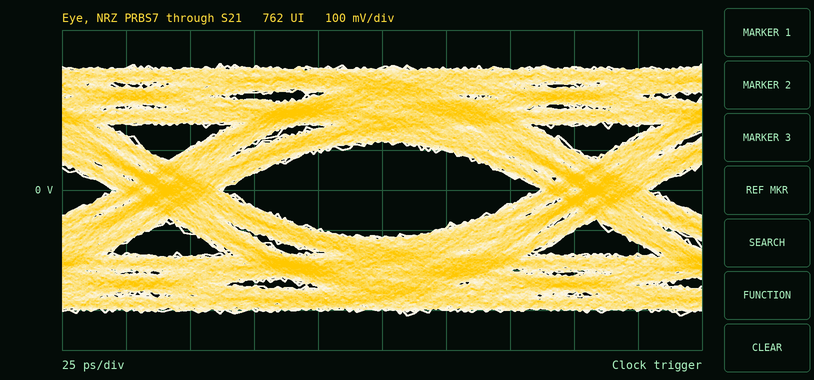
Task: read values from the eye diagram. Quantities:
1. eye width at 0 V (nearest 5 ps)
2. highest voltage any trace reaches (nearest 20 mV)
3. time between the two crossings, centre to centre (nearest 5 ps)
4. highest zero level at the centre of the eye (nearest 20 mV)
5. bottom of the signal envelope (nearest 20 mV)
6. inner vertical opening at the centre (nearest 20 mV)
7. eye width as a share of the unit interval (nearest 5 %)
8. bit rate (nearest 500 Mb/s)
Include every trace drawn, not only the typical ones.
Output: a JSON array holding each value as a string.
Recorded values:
["125 ps", "320 mV", "165 ps", "-120 mV", "-320 mV", "240 mV", "75 %", "6.0 Gb/s"]
